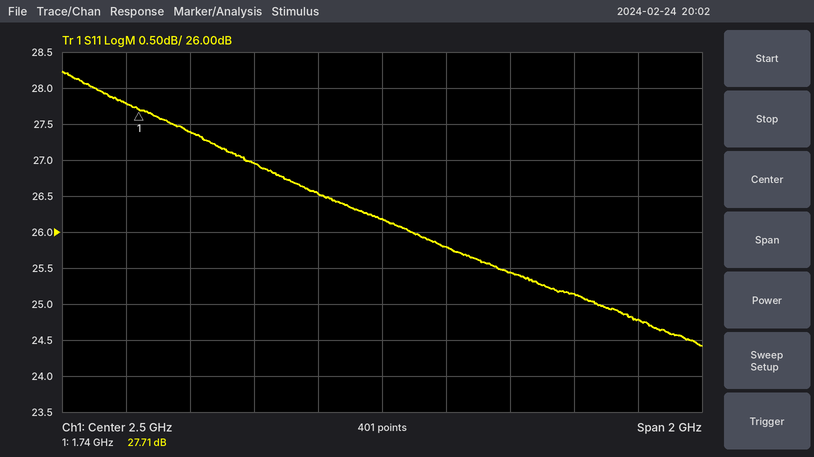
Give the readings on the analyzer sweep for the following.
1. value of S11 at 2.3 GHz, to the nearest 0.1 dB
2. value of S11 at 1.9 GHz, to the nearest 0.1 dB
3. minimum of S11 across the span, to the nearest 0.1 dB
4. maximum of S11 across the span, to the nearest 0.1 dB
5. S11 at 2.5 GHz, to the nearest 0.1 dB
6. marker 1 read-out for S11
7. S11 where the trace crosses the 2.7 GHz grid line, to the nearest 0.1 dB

26.5 dB
27.4 dB
24.4 dB
28.2 dB
26.2 dB
27.71 dB
25.8 dB
